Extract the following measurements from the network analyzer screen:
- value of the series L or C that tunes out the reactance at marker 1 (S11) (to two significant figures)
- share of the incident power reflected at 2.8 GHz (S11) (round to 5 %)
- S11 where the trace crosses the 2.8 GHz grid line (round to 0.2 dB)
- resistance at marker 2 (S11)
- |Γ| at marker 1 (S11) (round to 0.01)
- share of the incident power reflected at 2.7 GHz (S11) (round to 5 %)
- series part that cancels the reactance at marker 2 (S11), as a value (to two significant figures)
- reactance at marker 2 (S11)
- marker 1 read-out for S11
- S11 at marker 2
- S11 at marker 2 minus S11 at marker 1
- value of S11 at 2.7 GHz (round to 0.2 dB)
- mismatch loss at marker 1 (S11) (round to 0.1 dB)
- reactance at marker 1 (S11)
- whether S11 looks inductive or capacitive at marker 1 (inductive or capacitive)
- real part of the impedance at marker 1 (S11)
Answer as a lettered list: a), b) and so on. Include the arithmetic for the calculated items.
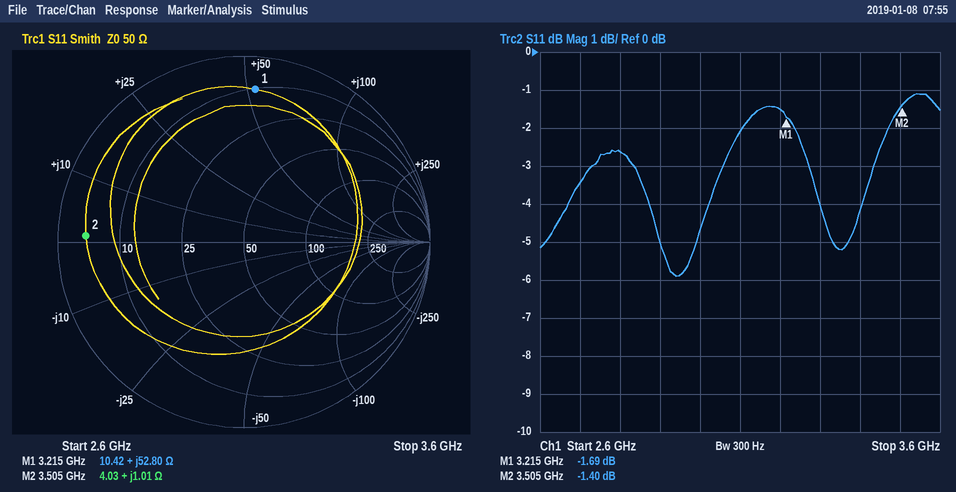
a) C = 1/(2π × 3.215 GHz × 52.8 Ω) ≈ 938 fF, so 940 fF to two significant figures
b) 10^(-2.6/10) ≈ 55 %
c) -2.6 dB
d) 4.03 Ω
e) 0.82
f) 10^(-3.4/10) ≈ 45.7 %, so 45 % to the nearest 5 %
g) C = 1/(2π × 3.505 GHz × 1.01 Ω) ≈ 45 pF
h) +1.01 Ω
i) -1.69 dB
j) -1.40 dB
k) -1.4 − (-1.69) = 0.29 dB
l) -3.4 dB
m) −10 log10(1 − 10^(-1.69/10)) ≈ 4.9 dB
n) +52.80 Ω
o) inductive
p) 10.42 Ω
